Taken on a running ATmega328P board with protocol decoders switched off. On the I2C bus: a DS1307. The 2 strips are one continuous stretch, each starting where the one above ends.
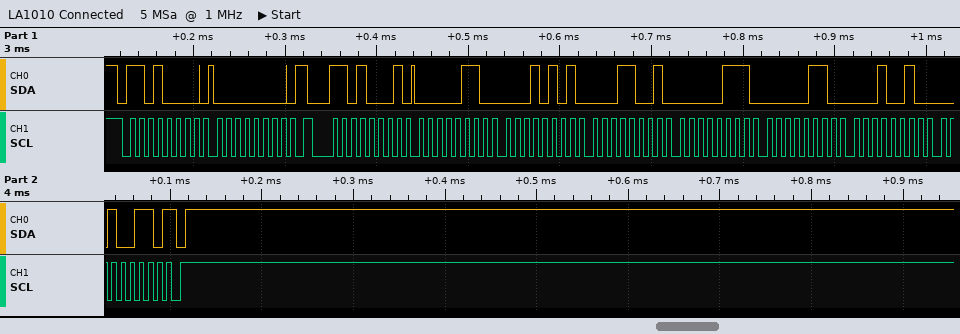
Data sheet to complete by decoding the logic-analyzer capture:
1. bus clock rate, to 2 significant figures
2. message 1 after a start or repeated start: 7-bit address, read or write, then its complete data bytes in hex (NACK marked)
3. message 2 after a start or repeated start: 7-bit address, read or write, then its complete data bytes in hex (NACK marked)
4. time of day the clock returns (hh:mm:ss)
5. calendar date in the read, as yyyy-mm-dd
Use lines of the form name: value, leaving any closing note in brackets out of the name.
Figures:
bus clock rate, to 2 significant figures: 100 kHz
message 1 after a start or repeated start: 7-bit address, read or write, then its complete data bytes in hex: 0x68 write: 00
message 2 after a start or repeated start: 7-bit address, read or write, then its complete data bytes in hex: 0x68 read: 06 15 19 07 06 12 26 NACK
time of day the clock returns: 19:15:06
calendar date in the read, as yyyy-mm-dd: 2026-12-06
